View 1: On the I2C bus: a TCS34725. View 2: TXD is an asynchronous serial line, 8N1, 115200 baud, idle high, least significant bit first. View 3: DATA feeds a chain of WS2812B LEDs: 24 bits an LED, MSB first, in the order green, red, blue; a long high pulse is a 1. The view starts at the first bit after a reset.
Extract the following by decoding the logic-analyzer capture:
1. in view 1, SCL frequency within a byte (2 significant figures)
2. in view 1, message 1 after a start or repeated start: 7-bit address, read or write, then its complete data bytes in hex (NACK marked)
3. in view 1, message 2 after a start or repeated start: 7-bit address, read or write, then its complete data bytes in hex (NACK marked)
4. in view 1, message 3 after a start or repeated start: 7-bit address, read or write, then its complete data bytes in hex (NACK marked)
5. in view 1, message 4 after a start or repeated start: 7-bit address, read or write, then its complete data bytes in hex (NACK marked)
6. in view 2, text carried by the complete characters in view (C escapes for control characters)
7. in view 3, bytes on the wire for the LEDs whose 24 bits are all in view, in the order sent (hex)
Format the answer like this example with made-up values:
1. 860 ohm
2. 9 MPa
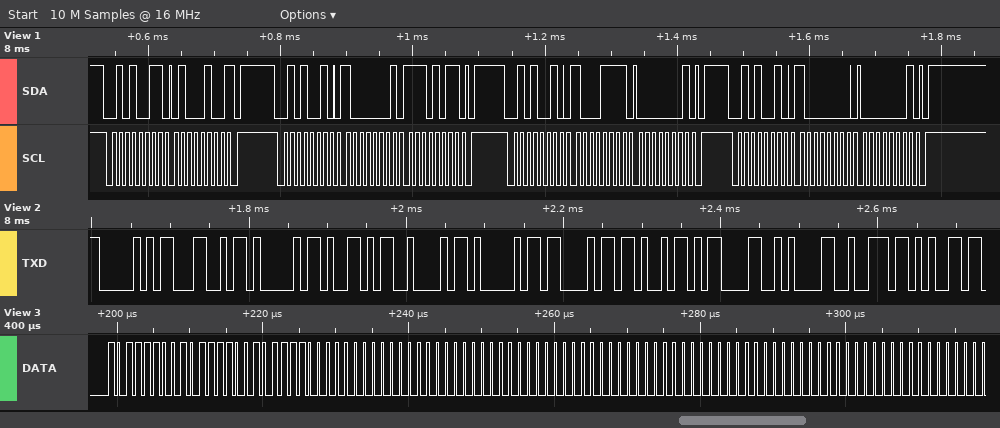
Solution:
1. 100 kHz
2. 0x29 read: 44 NACK
3. 0x29 write: 81 EB
4. 0x29 write: 8F 01
5. 0x29 write: 80 01
6. "PLAYBACK\r\nre"
7. BC BC BC 00 00 00 00 00 00 00 00 00
